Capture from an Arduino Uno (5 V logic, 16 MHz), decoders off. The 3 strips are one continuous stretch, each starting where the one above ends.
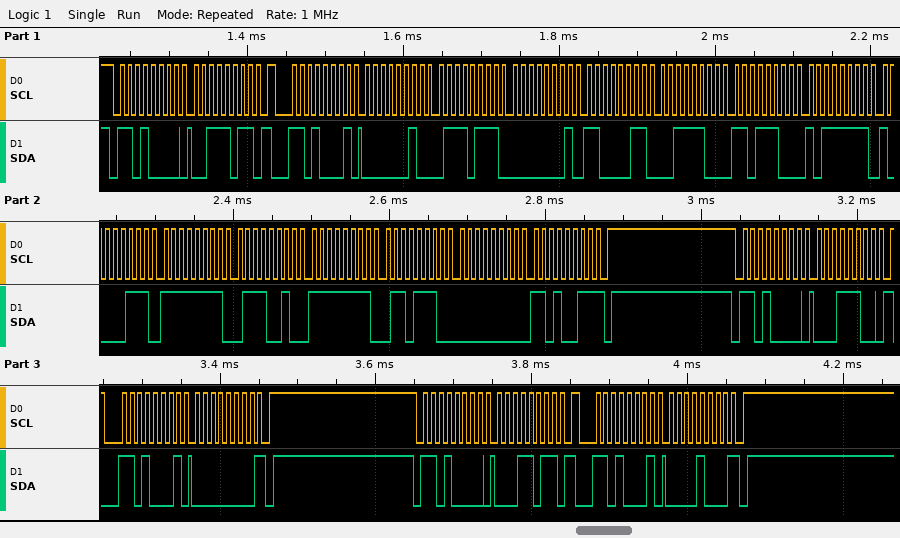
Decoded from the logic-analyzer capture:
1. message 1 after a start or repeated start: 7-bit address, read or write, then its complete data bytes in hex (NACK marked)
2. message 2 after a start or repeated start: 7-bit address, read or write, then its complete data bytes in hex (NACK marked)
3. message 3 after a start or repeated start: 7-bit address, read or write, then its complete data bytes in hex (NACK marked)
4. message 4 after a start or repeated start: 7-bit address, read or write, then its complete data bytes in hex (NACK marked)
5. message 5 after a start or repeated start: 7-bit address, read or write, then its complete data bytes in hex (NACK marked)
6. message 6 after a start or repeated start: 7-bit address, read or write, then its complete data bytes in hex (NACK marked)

0x68 write: 3B
0x68 read: 02 77 01 C3 3C DC BF 87 FF 72 FF 6E 00 D3 NACK
0x68 write: 1C
0x68 read: 00 NACK
0x68 write: 1B
0x68 read: 08 NACK
